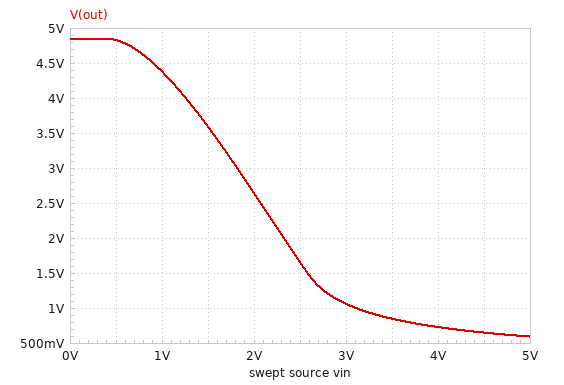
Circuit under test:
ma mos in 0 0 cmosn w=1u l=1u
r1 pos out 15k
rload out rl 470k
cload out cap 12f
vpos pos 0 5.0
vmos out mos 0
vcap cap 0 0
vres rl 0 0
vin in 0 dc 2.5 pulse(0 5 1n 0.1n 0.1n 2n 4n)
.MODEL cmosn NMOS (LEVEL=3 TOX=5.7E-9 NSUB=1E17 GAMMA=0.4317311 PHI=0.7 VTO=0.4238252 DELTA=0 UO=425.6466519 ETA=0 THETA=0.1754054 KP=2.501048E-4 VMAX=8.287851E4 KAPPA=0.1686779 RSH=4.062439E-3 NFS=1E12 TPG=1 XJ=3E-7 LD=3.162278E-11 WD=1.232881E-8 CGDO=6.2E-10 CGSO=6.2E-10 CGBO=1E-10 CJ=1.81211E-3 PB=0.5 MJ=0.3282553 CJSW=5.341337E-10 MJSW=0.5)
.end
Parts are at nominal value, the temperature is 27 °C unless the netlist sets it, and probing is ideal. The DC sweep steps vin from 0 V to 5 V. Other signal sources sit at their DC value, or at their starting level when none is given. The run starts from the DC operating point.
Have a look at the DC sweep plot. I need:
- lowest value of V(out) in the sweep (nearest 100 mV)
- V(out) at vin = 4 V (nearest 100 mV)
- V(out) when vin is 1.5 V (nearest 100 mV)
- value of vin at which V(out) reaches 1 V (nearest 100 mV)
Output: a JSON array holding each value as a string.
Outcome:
["600 mV", "700 mV", "3.6 V", "3.1 V"]
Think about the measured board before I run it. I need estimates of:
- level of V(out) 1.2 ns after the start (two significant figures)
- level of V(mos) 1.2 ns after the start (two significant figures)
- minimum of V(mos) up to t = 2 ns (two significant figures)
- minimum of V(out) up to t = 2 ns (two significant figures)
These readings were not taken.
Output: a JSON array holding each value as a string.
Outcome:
["860 mV", "860 mV", "590 mV", "590 mV"]
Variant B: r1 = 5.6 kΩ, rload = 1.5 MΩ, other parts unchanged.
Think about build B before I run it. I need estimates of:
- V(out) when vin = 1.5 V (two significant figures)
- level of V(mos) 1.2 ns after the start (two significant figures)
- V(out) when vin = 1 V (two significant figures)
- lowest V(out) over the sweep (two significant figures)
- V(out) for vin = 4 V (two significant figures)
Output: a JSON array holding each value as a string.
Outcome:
["4.5 V", "2.0 V", "4.8 V", "1.8 V", "2.4 V"]
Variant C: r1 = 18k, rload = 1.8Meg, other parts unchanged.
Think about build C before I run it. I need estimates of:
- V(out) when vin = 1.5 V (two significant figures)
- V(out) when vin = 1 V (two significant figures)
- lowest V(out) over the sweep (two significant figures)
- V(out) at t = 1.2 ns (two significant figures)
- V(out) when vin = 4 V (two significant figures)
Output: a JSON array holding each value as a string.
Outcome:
["3.4 V", "4.4 V", "490 mV", "770 mV", "590 mV"]
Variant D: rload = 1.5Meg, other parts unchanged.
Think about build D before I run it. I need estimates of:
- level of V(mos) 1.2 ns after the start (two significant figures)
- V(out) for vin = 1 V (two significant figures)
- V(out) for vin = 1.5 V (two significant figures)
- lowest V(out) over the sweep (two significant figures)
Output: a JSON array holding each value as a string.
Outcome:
["890 mV", "4.5 V", "3.7 V", "590 mV"]
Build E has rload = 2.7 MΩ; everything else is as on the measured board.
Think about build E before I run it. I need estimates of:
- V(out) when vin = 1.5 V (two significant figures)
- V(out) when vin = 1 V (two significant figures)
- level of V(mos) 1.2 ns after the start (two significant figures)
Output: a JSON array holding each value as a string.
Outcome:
["3.7 V", "4.5 V", "890 mV"]
